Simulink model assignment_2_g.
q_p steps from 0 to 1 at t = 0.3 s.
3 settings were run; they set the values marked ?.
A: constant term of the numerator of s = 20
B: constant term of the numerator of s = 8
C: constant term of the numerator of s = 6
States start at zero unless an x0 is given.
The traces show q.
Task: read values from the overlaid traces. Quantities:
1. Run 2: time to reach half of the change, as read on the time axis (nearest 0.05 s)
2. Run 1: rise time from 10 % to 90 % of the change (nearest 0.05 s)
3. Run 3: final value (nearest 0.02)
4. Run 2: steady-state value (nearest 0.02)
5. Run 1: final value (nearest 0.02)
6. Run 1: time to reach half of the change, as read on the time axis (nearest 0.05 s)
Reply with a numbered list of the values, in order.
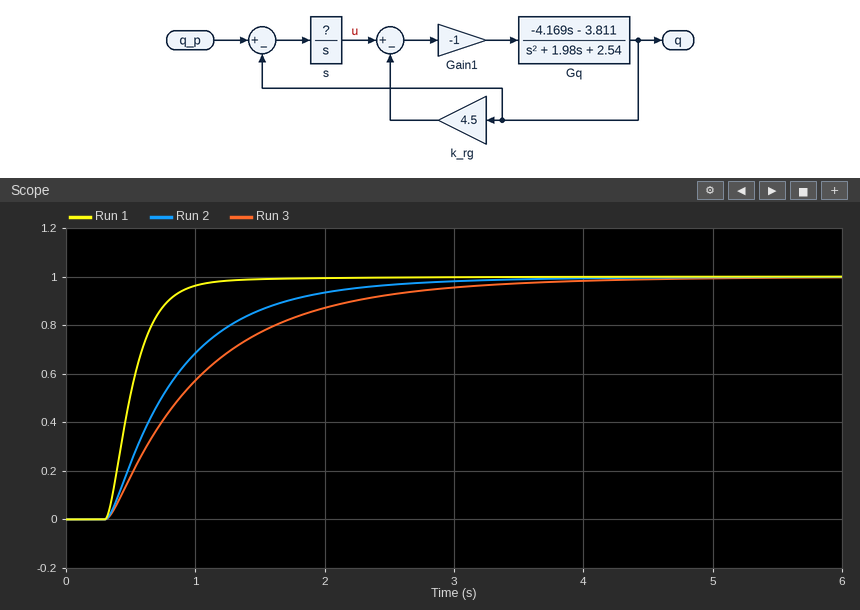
1. 0.75 s
2. 0.45 s
3. 1.00
4. 1.00
5. 1.00
6. 0.50 s
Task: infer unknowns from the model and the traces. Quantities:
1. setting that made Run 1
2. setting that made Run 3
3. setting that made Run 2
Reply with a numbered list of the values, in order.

1. A
2. C
3. B
